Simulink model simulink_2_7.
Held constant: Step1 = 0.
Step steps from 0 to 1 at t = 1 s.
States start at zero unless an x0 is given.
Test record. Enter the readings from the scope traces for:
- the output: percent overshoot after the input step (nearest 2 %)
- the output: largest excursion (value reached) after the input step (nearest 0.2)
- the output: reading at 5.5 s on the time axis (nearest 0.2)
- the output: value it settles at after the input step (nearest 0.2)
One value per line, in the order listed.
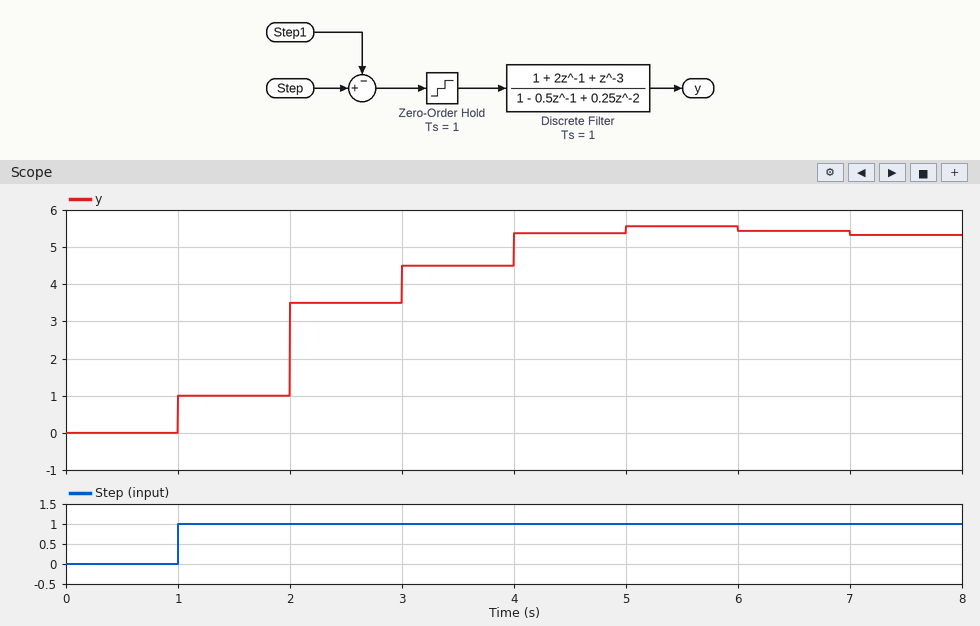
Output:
4 %
5.6
5.6
5.4
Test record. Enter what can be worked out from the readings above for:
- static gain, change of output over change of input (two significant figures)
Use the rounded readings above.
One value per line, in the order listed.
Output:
5.4
